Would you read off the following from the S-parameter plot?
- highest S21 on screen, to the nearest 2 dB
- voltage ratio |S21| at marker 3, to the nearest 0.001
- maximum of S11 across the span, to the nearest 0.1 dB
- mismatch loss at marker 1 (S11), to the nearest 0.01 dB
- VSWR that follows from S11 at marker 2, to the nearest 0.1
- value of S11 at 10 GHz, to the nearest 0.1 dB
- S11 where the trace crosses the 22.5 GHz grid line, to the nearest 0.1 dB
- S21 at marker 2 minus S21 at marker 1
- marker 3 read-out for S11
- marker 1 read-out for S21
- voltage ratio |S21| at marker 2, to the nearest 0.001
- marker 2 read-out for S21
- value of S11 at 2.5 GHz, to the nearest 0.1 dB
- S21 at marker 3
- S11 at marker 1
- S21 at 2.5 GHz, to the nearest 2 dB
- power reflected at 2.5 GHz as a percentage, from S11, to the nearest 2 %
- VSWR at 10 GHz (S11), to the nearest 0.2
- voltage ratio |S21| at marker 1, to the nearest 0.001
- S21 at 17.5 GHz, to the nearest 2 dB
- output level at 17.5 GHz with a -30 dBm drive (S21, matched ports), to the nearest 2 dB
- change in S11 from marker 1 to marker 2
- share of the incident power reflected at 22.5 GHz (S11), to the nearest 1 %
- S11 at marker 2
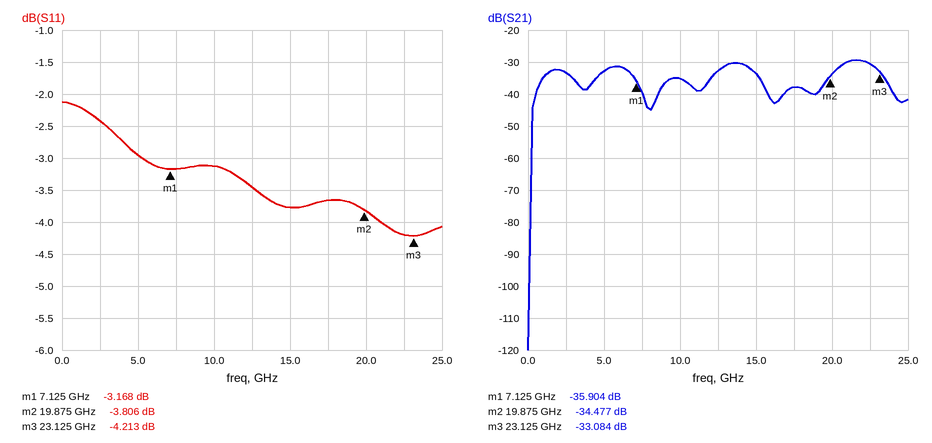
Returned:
-30 dB
0.022
-2.1 dB
2.86 dB
4.6
-3.1 dB
-4.2 dB
1.427 dB
-4.213 dB
-35.904 dB
0.019
-34.477 dB
-2.4 dB
-33.084 dB
-3.168 dB
-34 dB
58 %
5.6
0.016
-38 dB
-68 dBm
-0.638 dB
38 %
-3.806 dB
